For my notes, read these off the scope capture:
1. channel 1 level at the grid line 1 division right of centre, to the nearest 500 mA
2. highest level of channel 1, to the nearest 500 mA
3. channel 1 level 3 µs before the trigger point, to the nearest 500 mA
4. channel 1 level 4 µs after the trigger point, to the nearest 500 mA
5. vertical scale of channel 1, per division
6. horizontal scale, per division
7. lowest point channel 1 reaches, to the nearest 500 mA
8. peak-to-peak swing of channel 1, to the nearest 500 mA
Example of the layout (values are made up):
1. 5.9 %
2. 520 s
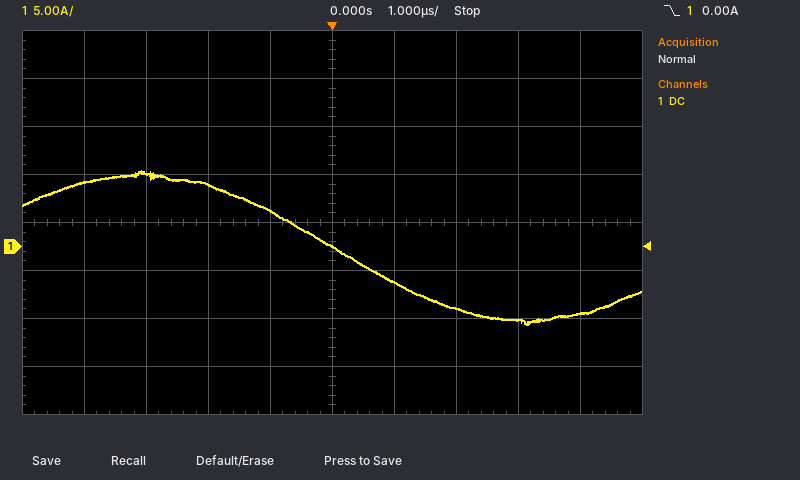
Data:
1. -3.5 A
2. 8.0 A
3. 7.5 A
4. -7.0 A
5. 5 A
6. 1 µs
7. -8.0 A
8. 16.0 A
